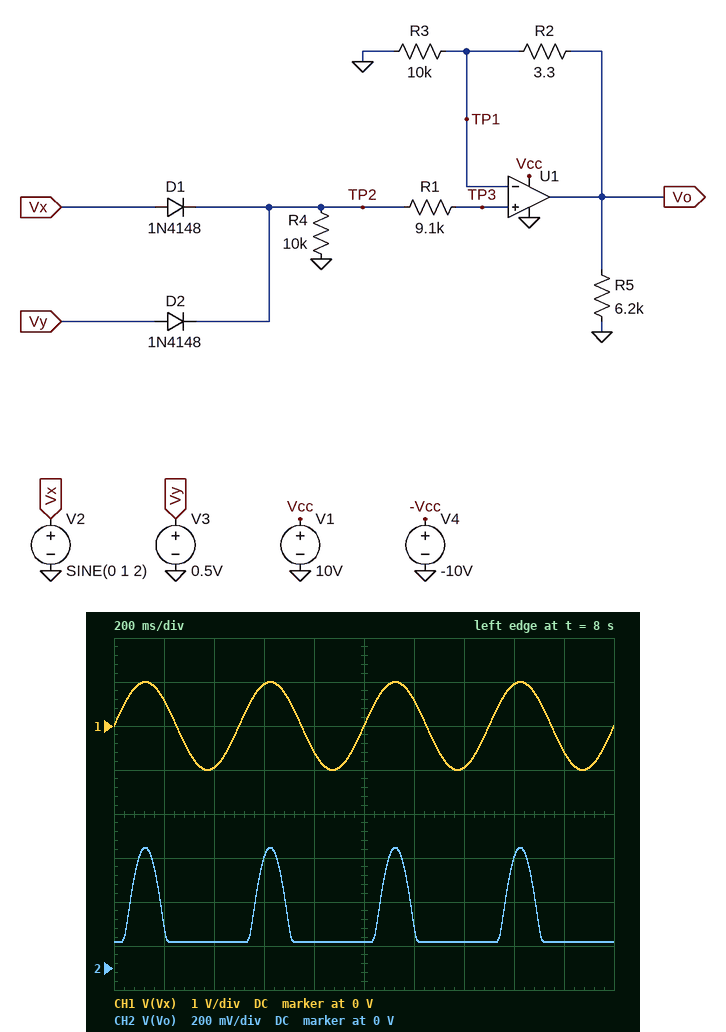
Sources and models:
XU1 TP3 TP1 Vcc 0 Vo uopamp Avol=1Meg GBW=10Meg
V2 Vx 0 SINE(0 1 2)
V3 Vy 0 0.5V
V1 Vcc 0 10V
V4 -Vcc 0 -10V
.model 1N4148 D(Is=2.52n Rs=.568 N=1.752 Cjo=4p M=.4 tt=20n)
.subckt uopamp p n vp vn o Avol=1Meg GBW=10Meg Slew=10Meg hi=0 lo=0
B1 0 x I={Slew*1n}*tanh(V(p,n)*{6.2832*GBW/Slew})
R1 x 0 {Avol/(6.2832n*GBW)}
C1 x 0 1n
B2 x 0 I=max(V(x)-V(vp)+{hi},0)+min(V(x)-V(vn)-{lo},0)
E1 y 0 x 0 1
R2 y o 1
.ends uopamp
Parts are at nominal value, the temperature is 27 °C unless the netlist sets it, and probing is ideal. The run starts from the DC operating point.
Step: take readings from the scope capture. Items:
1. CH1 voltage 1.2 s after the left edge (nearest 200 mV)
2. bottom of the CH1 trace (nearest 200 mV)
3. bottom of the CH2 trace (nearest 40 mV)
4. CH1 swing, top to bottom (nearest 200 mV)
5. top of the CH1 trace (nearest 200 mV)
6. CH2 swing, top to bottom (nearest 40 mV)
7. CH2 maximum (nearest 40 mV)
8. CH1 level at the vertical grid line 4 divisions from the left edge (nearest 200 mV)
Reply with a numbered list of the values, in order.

1. 600 mV
2. -1.0 V
3. 120 mV
4. 2.0 V
5. 1.0 V
6. 440 mV
7. 560 mV
8. -600 mV
